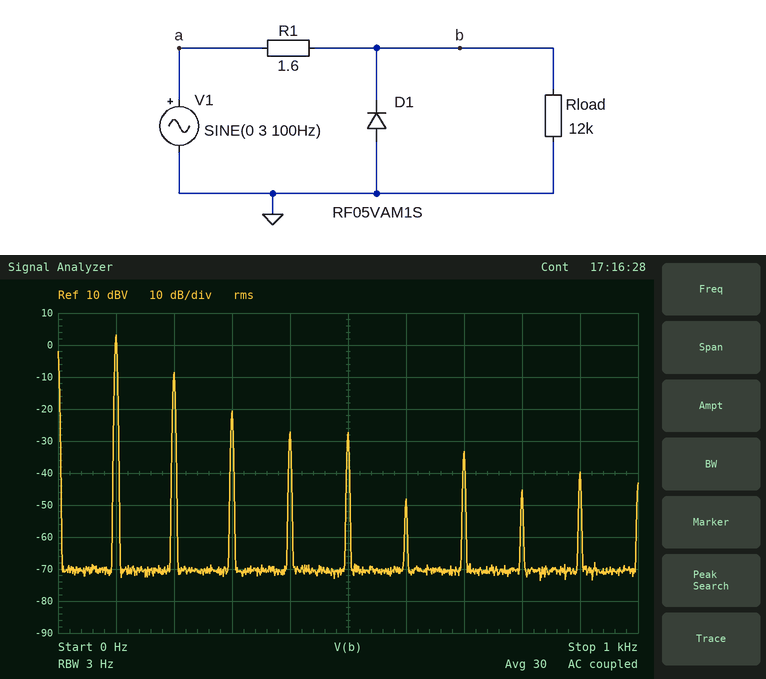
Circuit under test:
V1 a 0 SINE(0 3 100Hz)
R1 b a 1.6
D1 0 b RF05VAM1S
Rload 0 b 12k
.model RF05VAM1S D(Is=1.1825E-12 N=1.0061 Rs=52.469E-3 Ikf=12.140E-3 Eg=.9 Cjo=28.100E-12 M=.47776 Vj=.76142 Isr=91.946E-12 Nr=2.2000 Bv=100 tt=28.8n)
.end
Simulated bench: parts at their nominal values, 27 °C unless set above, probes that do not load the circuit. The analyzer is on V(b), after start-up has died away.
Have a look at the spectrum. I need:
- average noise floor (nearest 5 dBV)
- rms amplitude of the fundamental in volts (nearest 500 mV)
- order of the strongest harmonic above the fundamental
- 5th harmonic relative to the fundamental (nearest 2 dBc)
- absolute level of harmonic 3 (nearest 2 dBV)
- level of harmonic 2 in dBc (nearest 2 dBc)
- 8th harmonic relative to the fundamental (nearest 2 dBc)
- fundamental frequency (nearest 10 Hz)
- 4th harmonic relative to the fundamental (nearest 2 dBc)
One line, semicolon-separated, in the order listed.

-70 dBV; 1.5 V; 2; -30 dBc; -20 dBV; -12 dBc; -48 dBc; 100 Hz; -30 dBc
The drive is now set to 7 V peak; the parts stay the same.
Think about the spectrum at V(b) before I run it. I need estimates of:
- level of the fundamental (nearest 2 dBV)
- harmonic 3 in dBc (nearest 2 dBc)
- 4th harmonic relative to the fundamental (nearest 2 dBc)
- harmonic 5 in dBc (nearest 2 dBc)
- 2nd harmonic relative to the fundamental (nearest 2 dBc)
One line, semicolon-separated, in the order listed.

10 dBV; -28 dBc; -24 dBc; -34 dBc; -10 dBc
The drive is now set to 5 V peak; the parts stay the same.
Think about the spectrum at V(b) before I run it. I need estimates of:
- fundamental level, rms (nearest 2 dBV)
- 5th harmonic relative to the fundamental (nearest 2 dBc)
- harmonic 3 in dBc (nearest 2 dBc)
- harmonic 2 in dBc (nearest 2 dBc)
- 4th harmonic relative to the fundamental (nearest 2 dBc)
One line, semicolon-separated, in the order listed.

6 dBV; -32 dBc; -26 dBc; -10 dBc; -26 dBc
